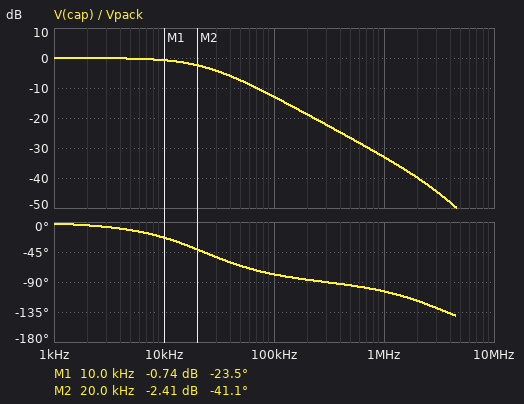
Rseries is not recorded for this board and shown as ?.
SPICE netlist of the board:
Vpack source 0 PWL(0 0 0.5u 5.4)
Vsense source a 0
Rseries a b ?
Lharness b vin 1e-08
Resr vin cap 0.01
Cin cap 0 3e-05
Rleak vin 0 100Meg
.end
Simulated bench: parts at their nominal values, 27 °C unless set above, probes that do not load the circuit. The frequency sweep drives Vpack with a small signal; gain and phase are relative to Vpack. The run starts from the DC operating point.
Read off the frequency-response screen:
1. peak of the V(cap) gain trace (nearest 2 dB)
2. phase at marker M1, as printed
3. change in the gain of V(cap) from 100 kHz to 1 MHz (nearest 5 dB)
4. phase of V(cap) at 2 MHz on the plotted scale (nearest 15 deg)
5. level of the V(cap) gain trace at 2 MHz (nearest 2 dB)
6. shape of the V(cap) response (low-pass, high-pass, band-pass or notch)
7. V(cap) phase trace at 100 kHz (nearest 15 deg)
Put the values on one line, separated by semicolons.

0 dB; -23.5 deg; -20 dB; -120 deg; -40 dB; low-pass; -75 deg
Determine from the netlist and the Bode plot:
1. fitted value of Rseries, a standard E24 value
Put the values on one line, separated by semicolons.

0.22 Ω
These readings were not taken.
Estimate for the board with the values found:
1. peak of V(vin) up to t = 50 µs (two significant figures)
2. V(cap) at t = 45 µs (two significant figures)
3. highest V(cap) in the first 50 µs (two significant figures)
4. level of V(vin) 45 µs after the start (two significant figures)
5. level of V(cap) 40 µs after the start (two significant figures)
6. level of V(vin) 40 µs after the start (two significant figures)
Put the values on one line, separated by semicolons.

5.4 V; 5.4 V; 5.4 V; 5.4 V; 5.4 V; 5.4 V
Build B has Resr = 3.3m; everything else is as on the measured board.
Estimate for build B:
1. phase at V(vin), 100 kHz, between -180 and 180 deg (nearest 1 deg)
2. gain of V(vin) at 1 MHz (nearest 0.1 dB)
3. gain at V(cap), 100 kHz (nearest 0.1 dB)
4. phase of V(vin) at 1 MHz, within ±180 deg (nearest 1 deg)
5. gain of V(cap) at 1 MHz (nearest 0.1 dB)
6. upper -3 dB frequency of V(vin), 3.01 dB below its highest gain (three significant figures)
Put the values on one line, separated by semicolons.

-75 deg; -31.3 dB; -12.7 dB; -73 deg; -32.8 dB; 23.9 kHz
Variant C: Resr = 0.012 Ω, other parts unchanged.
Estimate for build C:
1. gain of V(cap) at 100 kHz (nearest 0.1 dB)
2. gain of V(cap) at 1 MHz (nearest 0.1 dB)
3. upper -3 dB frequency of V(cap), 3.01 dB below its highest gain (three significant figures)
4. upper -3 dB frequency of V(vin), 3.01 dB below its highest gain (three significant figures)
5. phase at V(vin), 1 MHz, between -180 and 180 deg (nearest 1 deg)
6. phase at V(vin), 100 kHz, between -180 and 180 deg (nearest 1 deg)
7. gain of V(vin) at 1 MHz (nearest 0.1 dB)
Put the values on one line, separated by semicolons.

-13.0 dB; -33.1 dB; 23.0 kHz; 23.1 kHz; -38 deg; -66 deg; -25.2 dB
